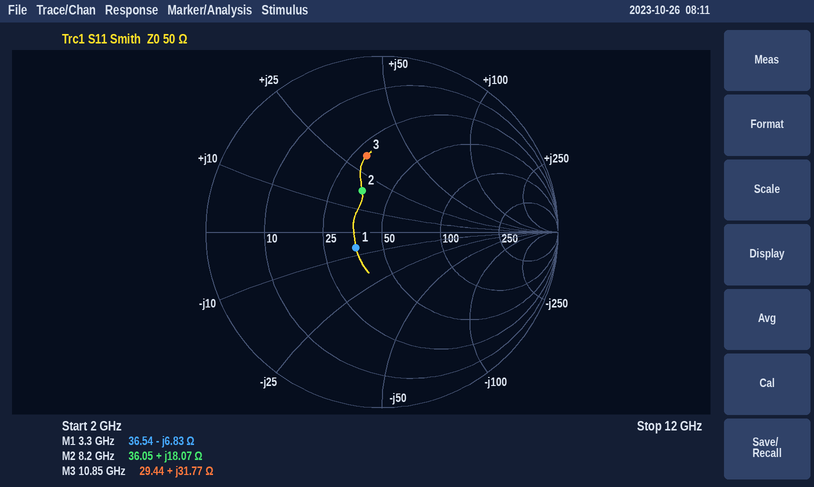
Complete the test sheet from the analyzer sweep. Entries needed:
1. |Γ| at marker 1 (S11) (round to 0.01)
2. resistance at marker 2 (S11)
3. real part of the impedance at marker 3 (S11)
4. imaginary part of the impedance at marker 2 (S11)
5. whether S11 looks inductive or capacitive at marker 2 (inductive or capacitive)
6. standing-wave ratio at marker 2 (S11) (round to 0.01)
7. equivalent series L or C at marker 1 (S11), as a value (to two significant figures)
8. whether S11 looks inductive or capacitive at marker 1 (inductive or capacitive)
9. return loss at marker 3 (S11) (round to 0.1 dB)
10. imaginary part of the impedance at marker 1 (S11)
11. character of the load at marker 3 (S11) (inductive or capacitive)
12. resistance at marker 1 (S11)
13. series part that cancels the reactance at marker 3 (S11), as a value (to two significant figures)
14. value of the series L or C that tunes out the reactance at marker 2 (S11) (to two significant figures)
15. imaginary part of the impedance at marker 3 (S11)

0.17
36.05 Ω
29.44 Ω
+18.07 Ω
inductive
1.70
7.1 pF
capacitive
7.1 dB
-6.83 Ω
inductive
36.54 Ω
460 fF
1.1 pF
+31.77 Ω
